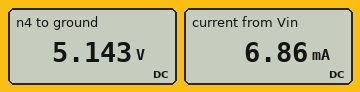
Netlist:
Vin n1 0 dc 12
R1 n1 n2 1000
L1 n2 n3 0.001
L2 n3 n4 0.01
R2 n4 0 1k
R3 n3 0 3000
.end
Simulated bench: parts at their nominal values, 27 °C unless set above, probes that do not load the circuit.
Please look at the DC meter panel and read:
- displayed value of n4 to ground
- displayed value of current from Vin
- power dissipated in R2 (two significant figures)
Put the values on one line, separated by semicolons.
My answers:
5.143 V; 6.86 mA; 26 mW
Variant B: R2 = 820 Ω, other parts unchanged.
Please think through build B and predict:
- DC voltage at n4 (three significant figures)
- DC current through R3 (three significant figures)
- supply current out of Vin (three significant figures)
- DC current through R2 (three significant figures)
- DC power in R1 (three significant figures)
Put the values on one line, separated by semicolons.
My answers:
4.70 V; 1.57 mA; 7.30 mA; 5.73 mA; 53.3 mW
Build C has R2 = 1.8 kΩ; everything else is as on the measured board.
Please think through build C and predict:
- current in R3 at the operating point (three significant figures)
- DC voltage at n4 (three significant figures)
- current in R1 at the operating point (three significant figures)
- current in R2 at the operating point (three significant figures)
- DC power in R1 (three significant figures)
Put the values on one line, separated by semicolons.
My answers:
2.12 mA; 6.35 V; 5.65 mA; 3.53 mA; 31.9 mW
